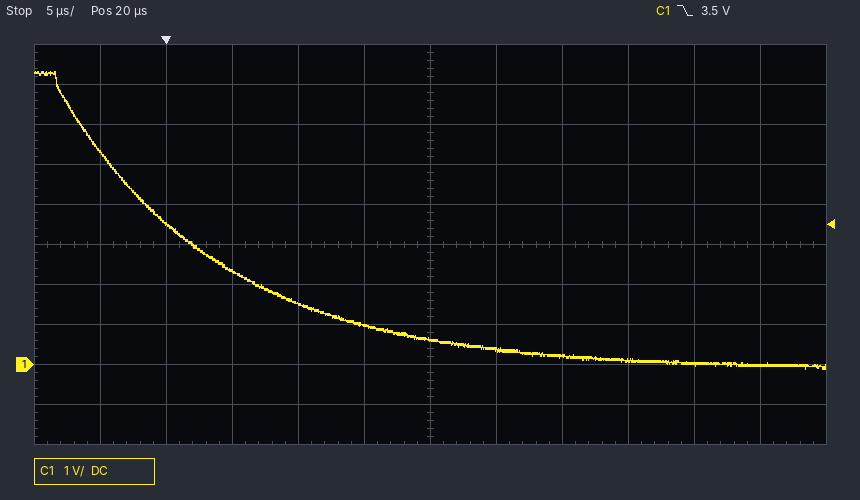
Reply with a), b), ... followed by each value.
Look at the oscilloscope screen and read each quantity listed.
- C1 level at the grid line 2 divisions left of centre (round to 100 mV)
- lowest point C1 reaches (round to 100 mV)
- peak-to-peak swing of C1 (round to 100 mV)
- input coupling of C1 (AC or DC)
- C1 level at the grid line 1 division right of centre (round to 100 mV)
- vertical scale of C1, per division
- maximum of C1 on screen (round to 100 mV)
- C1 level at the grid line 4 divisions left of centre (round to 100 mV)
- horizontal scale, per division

a) 1.5 V
b) -100 mV
c) 7.4 V
d) DC
e) 400 mV
f) 1 V
g) 7.3 V
h) 3.5 V
i) 5 µs
